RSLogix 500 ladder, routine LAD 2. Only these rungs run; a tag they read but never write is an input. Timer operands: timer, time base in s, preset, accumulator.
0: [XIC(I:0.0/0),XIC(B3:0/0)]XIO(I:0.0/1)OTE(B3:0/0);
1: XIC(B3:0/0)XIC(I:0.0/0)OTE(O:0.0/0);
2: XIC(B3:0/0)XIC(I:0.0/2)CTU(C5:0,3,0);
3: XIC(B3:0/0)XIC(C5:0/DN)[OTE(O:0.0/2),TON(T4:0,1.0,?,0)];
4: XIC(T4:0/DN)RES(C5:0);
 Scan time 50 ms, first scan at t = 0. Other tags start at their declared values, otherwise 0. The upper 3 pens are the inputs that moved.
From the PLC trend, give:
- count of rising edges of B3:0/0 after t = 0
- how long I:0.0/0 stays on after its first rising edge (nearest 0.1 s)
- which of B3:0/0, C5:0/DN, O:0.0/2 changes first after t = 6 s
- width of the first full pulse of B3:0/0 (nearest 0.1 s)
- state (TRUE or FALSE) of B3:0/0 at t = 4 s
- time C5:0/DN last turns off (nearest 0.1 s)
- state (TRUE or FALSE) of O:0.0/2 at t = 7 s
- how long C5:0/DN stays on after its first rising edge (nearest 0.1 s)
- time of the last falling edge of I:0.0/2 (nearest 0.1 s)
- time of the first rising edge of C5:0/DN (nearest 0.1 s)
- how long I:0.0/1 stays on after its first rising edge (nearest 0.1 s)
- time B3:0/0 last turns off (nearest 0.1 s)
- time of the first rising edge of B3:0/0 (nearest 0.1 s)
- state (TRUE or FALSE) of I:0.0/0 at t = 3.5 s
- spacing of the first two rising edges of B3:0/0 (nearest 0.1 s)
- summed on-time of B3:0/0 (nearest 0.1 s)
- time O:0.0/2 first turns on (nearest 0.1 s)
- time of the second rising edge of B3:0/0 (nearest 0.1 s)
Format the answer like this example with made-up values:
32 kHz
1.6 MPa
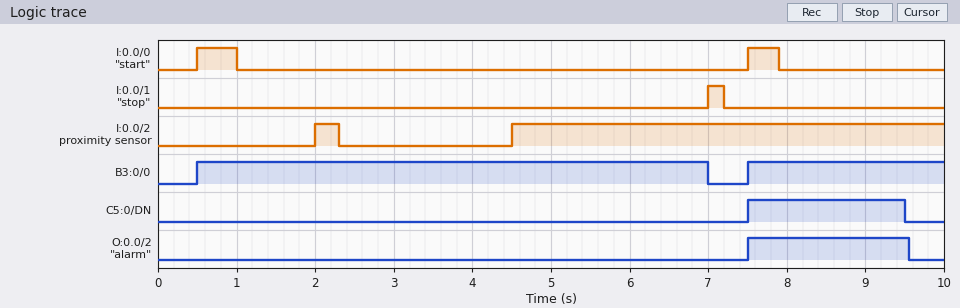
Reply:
2
0.5 s
B3:0/0
6.5 s
TRUE
9.5 s
FALSE
2.0 s
2.3 s
7.5 s
0.2 s
7.0 s
0.5 s
FALSE
7.0 s
9.0 s
7.5 s
7.5 s
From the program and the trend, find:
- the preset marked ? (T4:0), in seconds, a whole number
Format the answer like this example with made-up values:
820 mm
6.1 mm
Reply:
2 s
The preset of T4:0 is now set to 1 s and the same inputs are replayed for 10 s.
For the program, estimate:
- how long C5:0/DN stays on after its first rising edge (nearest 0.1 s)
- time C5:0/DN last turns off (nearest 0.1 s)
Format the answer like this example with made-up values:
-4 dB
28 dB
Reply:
1.0 s
8.5 s
